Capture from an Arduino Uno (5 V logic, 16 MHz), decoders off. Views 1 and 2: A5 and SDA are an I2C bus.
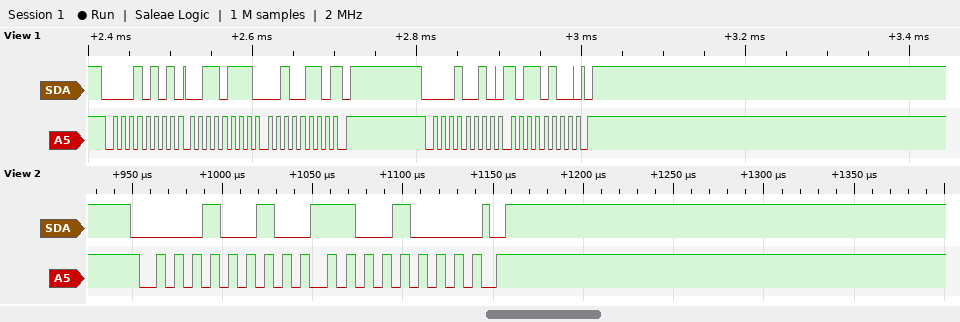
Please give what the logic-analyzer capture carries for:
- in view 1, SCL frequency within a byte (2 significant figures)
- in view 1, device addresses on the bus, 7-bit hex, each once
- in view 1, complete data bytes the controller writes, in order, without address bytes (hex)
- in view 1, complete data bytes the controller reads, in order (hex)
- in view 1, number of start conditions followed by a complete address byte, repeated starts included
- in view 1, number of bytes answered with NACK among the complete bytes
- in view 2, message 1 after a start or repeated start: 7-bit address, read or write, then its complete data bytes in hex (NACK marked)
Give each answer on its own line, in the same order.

100 kHz
0x0A 0x09
B4
37 26
2
1
0x09 write: C8
